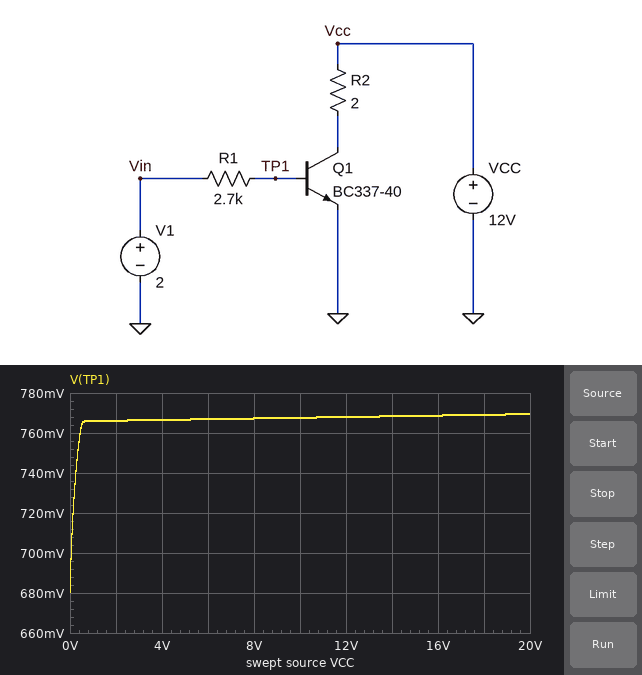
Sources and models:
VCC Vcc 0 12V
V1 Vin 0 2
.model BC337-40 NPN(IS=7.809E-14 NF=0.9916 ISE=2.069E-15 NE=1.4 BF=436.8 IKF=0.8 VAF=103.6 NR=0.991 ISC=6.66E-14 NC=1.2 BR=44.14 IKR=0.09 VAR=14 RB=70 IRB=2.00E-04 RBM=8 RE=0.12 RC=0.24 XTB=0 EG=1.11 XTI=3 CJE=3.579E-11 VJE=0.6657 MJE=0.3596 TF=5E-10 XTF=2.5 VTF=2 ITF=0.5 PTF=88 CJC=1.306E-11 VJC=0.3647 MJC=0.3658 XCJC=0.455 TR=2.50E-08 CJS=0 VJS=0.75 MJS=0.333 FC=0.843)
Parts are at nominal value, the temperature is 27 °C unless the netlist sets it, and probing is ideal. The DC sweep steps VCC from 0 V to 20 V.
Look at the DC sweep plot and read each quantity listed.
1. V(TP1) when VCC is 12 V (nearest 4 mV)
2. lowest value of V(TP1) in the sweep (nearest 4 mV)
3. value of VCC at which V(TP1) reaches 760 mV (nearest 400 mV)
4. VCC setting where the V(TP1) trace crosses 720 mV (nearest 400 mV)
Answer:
768 mV
680 mV
400 mV
0 V
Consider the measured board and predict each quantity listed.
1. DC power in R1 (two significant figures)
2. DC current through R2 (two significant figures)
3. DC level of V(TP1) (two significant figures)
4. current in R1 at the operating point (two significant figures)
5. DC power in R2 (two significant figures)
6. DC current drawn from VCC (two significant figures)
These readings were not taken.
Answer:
560 µW
170 mA
770 mV
460 µA
60 mW
170 mA
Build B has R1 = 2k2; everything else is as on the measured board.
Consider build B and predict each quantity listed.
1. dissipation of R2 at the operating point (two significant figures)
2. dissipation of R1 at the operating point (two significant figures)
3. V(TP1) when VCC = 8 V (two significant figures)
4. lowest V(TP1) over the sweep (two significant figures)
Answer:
84 mW
680 µW
780 mV
690 mV
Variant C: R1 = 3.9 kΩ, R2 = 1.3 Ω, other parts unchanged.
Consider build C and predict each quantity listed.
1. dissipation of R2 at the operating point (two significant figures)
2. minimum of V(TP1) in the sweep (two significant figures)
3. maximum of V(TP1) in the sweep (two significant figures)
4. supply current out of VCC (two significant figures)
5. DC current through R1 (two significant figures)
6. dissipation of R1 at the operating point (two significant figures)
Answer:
21 mW
670 mV
750 mV
130 mA
320 µA
400 µW
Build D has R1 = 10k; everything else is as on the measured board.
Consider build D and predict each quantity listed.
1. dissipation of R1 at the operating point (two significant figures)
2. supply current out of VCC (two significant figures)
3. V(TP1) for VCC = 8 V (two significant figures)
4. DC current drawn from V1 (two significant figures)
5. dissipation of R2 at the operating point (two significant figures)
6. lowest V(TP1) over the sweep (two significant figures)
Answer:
170 µW
56 mA
710 mV
130 µA
6.2 mW
640 mV
